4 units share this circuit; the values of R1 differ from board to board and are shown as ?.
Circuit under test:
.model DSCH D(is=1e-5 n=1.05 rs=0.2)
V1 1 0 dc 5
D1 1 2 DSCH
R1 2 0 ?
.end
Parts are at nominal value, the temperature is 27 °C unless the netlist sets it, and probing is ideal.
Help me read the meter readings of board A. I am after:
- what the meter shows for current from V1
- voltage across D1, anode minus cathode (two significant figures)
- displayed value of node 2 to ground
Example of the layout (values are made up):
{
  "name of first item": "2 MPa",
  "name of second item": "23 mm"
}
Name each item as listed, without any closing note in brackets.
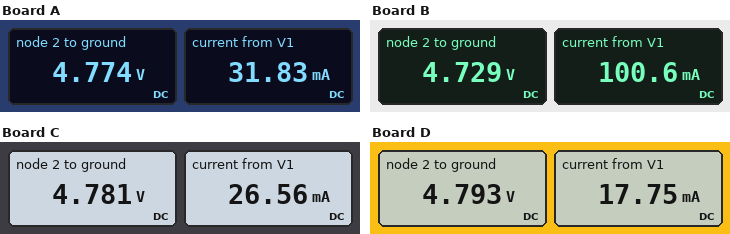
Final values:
{
  "what the meter shows for current from V1": "31.83 mA",
  "voltage across D1, anode minus cathode": "230 mV",
  "displayed value of node 2 to ground": "4.774 V"
}
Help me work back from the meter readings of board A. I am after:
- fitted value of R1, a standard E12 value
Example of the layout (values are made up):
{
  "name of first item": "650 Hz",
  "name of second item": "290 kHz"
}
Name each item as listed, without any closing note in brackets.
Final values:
{
  "fitted value of R1, a standard E12 value": "150 Ω"
}
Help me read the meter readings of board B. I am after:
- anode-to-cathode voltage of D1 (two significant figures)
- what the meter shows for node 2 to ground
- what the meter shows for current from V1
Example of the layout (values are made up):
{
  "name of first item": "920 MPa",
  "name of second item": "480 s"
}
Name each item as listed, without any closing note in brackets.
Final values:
{
  "anode-to-cathode voltage of D1": "270 mV",
  "what the meter shows for node 2 to ground": "4.729 V",
  "what the meter shows for current from V1": "100.6 mA"
}
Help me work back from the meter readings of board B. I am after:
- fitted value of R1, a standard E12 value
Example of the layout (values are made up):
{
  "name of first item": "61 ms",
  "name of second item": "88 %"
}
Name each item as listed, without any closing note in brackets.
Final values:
{
  "fitted value of R1, a standard E12 value": "47 Ω"
}
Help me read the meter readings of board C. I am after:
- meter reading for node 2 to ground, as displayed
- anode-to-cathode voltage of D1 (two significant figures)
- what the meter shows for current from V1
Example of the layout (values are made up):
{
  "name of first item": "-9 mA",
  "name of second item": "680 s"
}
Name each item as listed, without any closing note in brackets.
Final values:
{
  "meter reading for node 2 to ground, as displayed": "4.781 V",
  "anode-to-cathode voltage of D1": "220 mV",
  "what the meter shows for current from V1": "26.56 mA"
}
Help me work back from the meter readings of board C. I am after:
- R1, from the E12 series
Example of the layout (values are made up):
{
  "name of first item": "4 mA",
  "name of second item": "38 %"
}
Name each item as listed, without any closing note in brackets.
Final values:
{
  "R1, from the E12 series": "180 Ω"
}
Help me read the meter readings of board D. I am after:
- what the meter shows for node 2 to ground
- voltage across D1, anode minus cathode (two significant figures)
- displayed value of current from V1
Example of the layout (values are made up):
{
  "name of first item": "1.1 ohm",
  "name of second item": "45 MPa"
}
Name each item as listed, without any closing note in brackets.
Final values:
{
  "what the meter shows for node 2 to ground": "4.793 V",
  "voltage across D1, anode minus cathode": "210 mV",
  "displayed value of current from V1": "17.75 mA"
}
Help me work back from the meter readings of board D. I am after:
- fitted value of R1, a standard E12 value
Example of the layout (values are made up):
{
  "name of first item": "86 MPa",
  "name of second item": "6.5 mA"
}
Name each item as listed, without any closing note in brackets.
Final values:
{
  "fitted value of R1, a standard E12 value": "270 Ω"
}
